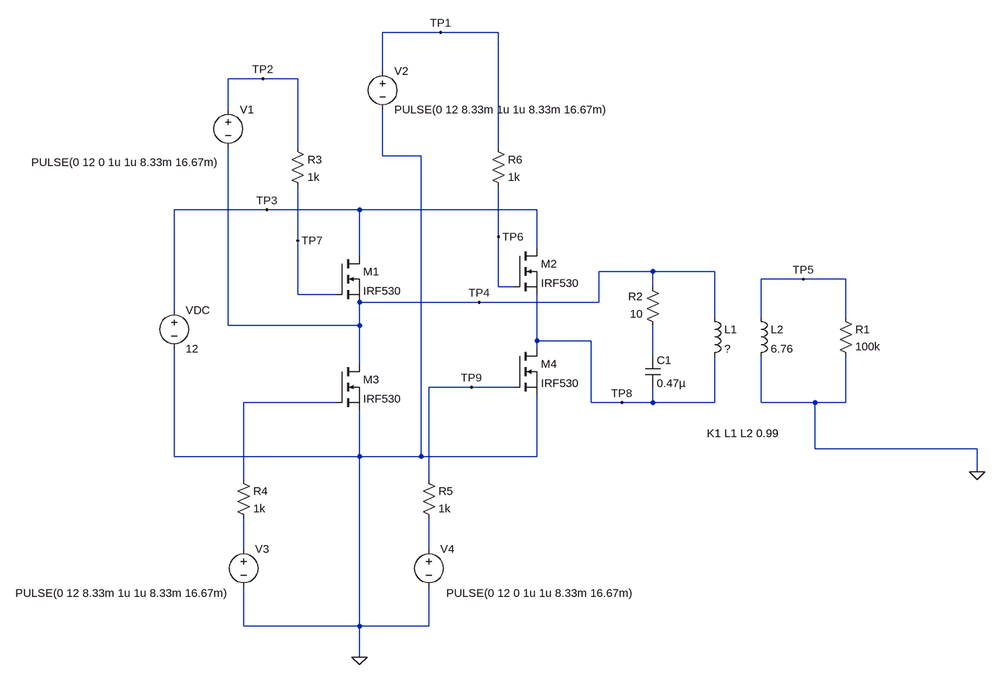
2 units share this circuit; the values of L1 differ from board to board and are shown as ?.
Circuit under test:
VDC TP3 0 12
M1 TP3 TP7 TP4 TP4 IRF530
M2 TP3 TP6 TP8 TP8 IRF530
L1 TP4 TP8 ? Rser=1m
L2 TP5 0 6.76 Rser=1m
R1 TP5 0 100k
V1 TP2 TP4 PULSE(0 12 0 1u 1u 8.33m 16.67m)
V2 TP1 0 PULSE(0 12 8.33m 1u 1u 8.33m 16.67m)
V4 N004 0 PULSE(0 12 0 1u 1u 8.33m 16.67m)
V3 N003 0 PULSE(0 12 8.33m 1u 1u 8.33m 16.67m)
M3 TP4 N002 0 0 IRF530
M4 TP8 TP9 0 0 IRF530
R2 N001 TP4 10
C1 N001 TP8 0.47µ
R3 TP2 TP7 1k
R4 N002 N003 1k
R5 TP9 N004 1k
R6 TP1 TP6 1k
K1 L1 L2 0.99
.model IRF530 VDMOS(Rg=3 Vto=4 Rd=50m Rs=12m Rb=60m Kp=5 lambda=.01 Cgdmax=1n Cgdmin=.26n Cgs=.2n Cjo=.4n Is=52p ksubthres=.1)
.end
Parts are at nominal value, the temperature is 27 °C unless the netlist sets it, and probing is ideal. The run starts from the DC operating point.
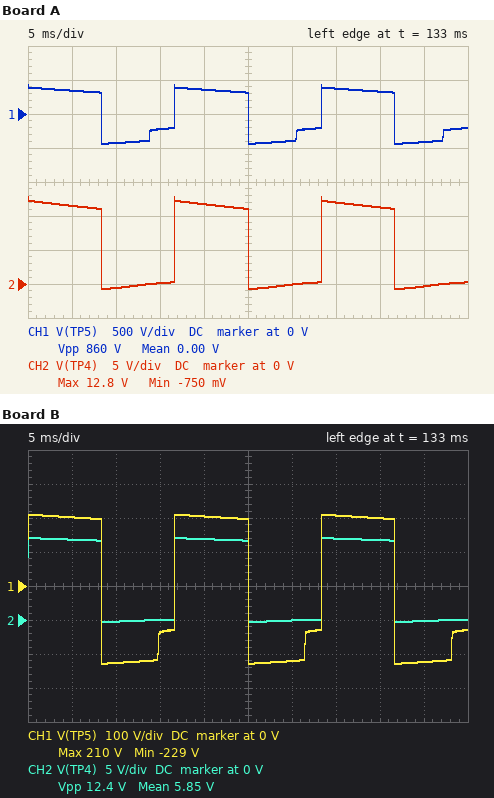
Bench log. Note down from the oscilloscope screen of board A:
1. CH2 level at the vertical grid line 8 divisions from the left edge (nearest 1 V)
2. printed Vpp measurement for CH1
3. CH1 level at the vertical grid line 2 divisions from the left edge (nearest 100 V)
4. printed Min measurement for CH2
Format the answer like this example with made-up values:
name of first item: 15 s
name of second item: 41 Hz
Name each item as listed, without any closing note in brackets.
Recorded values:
CH2 level at the vertical grid line 8 divisions from the left edge: 11 V
printed Vpp measurement for CH1: 860 V
CH1 level at the vertical grid line 2 divisions from the left edge: -400 V
printed Min measurement for CH2: -750 mV
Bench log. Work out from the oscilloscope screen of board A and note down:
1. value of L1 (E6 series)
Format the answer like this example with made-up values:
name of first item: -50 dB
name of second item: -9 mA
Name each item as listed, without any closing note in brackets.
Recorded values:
value of L1: 6.8 mH
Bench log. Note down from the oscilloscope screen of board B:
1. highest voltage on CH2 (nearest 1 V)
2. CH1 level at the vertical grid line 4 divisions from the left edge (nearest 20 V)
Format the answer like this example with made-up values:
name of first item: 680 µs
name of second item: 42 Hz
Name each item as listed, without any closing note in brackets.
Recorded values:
highest voltage on CH2: 12 V
CH1 level at the vertical grid line 4 divisions from the left edge: 200 V
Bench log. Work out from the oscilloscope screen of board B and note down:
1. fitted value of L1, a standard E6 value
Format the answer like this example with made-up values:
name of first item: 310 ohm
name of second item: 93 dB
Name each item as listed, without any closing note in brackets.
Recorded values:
fitted value of L1, a standard E6 value: 22 mH
